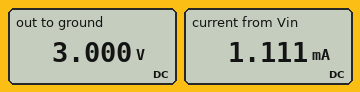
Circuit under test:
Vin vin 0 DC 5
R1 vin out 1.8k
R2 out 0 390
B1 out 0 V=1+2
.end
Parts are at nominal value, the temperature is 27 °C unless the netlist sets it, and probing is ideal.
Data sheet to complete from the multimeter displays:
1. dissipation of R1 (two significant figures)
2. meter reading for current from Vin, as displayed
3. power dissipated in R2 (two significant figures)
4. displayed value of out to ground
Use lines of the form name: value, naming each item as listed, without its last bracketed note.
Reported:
dissipation of R1: 2.2 mW
meter reading for current from Vin, as displayed: 1.111 mA
power dissipated in R2: 23 mW
displayed value of out to ground: 3.000 V
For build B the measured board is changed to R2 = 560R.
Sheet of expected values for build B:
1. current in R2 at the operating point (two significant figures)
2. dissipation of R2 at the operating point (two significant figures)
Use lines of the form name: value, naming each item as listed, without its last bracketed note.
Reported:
current in R2 at the operating point: 5.4 mA
dissipation of R2 at the operating point: 16 mW
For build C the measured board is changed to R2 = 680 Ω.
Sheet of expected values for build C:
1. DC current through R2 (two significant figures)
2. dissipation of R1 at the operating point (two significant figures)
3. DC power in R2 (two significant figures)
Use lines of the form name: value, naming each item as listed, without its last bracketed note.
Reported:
DC current through R2: 4.4 mA
dissipation of R1 at the operating point: 2.2 mW
DC power in R2: 13 mW
